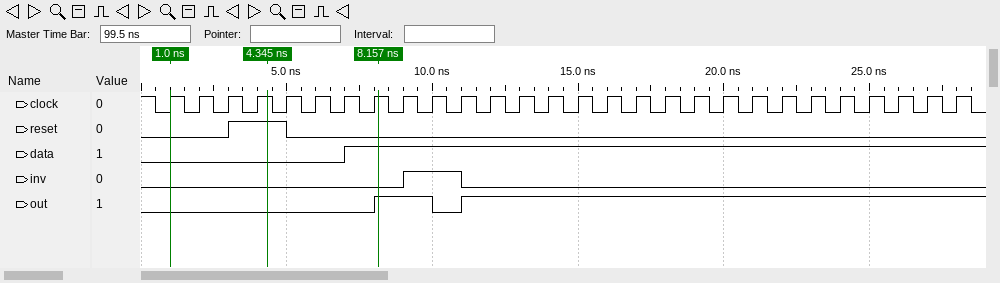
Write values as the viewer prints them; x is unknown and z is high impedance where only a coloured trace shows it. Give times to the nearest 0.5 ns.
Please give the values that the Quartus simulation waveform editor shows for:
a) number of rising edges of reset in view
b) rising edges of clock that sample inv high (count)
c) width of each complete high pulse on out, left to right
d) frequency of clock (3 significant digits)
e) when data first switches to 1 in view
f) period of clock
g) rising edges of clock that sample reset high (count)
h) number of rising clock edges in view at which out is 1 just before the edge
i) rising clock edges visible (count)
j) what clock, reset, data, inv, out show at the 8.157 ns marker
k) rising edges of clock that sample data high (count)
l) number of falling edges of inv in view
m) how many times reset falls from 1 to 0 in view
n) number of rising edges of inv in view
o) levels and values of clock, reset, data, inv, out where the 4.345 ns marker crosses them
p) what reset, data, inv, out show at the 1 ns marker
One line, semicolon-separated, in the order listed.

1; 2; 2 ns; 1.00 GHz; 7 ns; 1 ns; 2; 19; 28; clock=1, reset=0, data=1, inv=0, out=1; 21; 1; 1; 1; clock=1, reset=1, data=0, inv=0, out=0; reset=0, data=0, inv=0, out=0
